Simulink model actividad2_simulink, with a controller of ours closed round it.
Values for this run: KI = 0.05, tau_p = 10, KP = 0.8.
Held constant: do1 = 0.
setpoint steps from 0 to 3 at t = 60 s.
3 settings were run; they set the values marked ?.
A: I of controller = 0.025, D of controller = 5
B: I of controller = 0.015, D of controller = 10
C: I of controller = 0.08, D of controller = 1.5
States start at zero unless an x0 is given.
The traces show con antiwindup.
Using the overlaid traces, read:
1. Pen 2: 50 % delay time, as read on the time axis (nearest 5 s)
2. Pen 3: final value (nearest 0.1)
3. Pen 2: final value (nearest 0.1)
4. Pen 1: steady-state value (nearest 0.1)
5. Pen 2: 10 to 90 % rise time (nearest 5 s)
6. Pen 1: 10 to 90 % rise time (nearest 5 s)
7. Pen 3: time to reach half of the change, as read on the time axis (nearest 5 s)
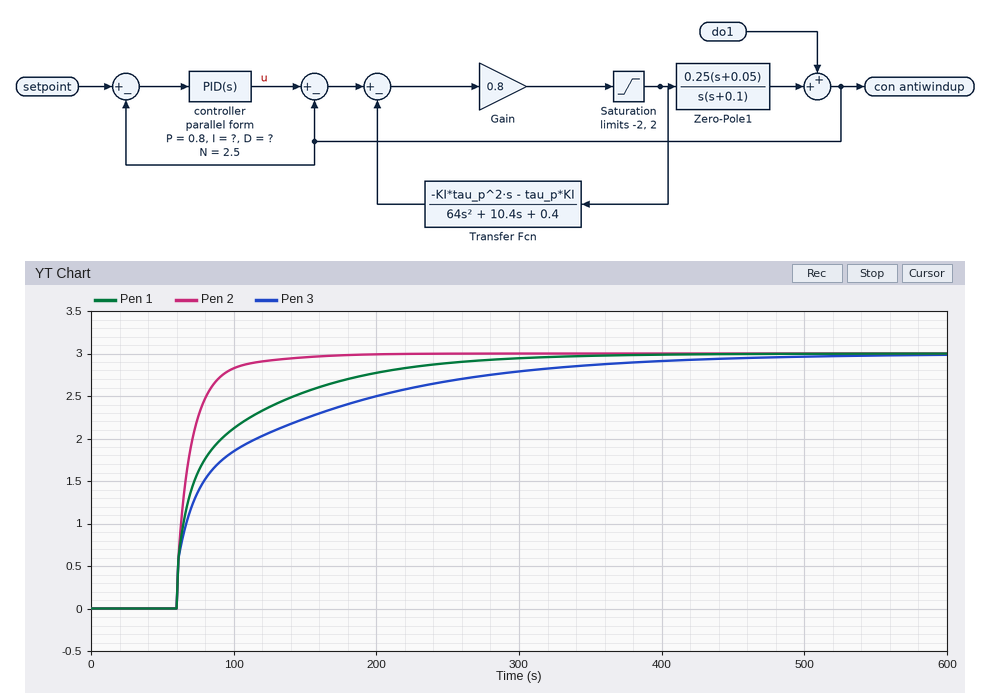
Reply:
65 s
3.0
3.0
3.0
30 s
120 s
80 s
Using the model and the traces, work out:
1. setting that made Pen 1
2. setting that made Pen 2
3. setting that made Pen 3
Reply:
A
C
B
